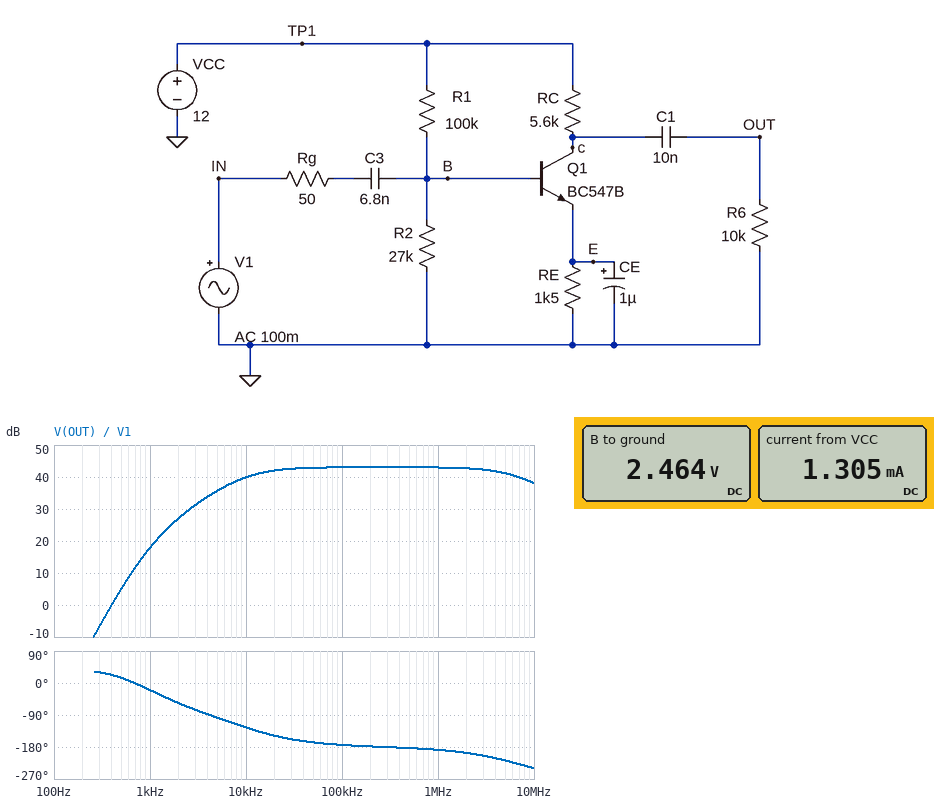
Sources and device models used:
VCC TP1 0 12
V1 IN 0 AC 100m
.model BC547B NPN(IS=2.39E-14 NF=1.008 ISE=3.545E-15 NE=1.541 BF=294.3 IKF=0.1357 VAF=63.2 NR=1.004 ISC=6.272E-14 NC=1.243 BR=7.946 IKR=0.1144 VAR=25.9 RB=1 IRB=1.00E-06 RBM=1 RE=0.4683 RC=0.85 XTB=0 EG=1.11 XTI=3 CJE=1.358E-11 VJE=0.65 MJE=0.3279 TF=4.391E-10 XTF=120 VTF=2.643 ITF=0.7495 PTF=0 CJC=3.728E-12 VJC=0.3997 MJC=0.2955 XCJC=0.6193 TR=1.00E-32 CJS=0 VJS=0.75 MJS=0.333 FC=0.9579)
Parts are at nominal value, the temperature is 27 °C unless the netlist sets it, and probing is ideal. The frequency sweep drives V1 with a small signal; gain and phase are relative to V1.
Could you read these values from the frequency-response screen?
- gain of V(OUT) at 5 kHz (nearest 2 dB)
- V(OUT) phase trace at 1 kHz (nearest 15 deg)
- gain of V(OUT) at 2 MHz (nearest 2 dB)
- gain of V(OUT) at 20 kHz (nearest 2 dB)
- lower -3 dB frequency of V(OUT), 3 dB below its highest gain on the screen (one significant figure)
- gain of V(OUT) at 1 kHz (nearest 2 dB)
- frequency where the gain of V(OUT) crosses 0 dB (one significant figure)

36 dB
-15 deg
42 dB
42 dB
10 kHz
18 dB
400 Hz
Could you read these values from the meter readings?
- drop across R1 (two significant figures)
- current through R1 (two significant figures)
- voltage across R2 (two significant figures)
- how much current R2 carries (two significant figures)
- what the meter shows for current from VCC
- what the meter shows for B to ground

9.5 V
95 µA
2.5 V
91 µA
1.305 mA
2.464 V
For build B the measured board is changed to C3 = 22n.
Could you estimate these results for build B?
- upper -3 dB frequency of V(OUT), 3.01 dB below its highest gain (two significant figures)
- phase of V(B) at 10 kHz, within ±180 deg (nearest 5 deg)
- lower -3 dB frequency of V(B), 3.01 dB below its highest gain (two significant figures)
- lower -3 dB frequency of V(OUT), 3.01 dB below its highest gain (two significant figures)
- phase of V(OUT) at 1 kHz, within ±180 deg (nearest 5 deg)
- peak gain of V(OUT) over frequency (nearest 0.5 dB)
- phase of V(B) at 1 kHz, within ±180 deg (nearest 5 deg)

6.6 MHz
5 deg
420 Hz
8.0 kHz
-40 deg
43.5 dB
20 deg
